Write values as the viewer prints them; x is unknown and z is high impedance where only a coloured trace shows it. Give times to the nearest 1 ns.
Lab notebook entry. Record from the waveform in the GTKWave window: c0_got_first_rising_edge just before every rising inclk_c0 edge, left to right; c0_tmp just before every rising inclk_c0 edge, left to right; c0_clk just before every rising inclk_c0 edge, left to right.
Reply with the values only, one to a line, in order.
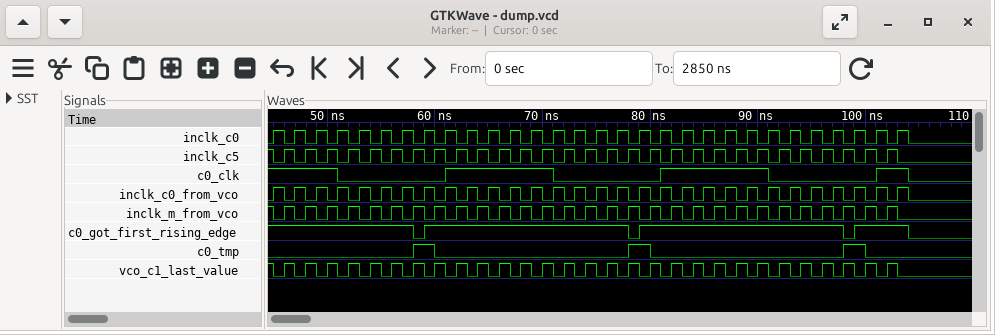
1 1 1 1 1 1 1 0 1 1 1 1 1 1 1 1 1 0 1 1 1 1 1 1 1 1 1 0 1 1
0 0 0 0 0 0 0 1 0 0 0 0 0 0 0 0 0 1 0 0 0 0 0 0 0 0 0 1 0 0
1 1 1 1 0 0 0 0 0 1 1 1 1 1 0 0 0 0 0 1 1 1 1 1 0 0 0 0 0 1
